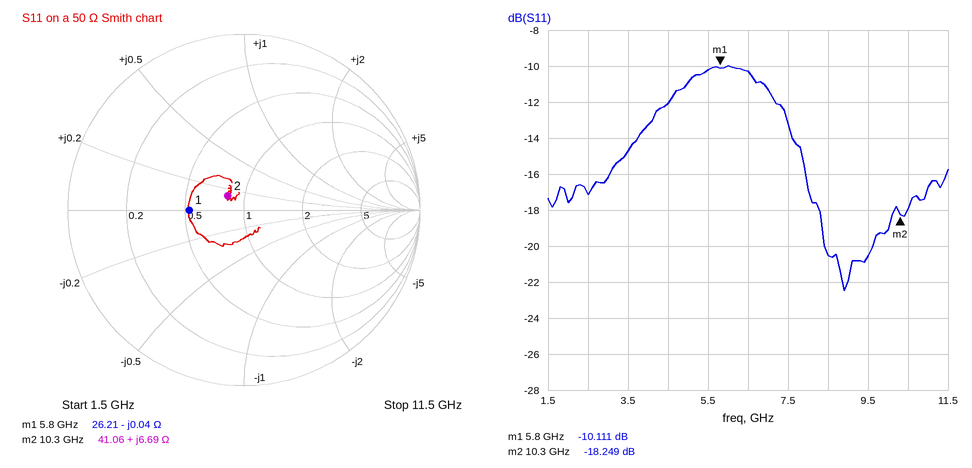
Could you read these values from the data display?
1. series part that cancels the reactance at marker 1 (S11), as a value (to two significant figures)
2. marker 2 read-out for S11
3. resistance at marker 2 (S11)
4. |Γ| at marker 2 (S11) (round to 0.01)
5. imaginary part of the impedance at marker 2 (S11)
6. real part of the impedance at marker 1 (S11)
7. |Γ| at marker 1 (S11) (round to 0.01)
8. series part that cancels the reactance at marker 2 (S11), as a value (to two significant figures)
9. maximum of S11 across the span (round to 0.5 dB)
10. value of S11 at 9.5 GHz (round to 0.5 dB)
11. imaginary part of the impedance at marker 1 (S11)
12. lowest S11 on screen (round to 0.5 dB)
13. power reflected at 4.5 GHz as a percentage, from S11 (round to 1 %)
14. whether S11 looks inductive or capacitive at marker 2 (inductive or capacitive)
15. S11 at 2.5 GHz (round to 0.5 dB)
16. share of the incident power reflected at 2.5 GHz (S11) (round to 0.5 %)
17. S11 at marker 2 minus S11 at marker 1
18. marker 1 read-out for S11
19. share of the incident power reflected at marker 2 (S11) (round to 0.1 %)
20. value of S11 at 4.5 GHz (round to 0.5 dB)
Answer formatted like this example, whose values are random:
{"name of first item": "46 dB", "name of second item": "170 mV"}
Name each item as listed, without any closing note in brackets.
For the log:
{"series part that cancels the reactance at marker 1 (S11), as a value": "1.1 pH", "marker 2 read-out for S11": "-18.249 dB", "resistance at marker 2": "41.06 Ω", "|Γ| at marker 2 (S11)": "0.12", "imaginary part of the impedance at marker 2": "+6.69 Ω", "real part of the impedance at marker 1": "26.21 Ω", "|Γ| at marker 1 (S11)": "0.31", "series part that cancels the reactance at marker 2 (S11), as a value": "2.3 pF", "maximum of S11 across the span": "-10.0 dB", "value of S11 at 9.5 GHz": "-20.5 dB", "imaginary part of the impedance at marker 1": "-0.04 Ω", "lowest S11 on screen": "-22.5 dB", "power reflected at 4.5 GHz as a percentage, from S11": "6 %", "whether S11 looks inductive or capacitive at marker 2": "inductive", "S11 at 2.5 GHz": "-17.0 dB", "share of the incident power reflected at 2.5 GHz (S11)": "2.0 %", "S11 at marker 2 minus S11 at marker 1": "-8.138 dB", "marker 1 read-out for S11": "-10.111 dB", "share of the incident power reflected at marker 2 (S11)": "1.5 %", "value of S11 at 4.5 GHz": "-12.0 dB"}
